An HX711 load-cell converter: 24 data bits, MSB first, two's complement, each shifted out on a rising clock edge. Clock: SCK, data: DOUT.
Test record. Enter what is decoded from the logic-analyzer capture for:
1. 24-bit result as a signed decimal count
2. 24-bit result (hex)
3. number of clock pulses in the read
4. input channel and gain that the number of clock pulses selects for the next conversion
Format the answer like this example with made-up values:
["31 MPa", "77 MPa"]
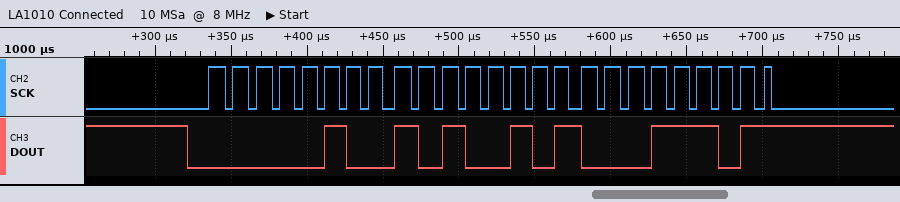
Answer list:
["304413", "0x04A51D", "25", "channel A, gain 128"]
